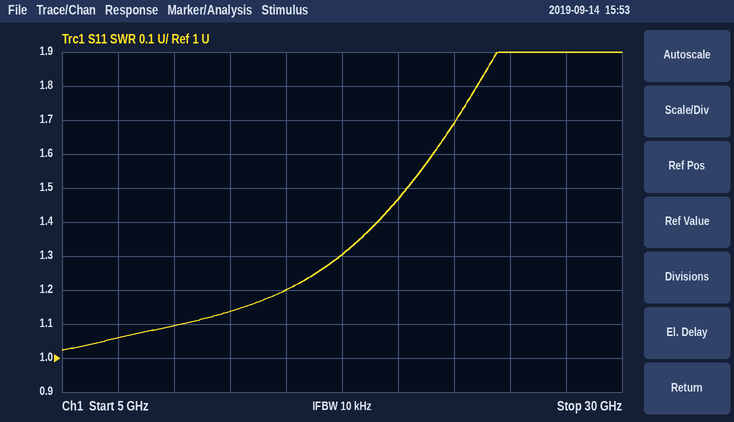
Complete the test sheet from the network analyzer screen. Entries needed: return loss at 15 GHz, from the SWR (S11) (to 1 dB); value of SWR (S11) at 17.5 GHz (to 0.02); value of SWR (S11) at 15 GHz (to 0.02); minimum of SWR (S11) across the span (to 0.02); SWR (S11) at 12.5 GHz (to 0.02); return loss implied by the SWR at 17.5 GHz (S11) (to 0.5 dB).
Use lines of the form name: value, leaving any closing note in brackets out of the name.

return loss at 15 GHz, from the SWR (S11): 21 dB
value of SWR (S11) at 17.5 GHz: 1.30
value of SWR (S11) at 15 GHz: 1.20
minimum of SWR (S11) across the span: 1.02
SWR (S11) at 12.5 GHz: 1.14
return loss implied by the SWR at 17.5 GHz (S11): 17.5 dB
